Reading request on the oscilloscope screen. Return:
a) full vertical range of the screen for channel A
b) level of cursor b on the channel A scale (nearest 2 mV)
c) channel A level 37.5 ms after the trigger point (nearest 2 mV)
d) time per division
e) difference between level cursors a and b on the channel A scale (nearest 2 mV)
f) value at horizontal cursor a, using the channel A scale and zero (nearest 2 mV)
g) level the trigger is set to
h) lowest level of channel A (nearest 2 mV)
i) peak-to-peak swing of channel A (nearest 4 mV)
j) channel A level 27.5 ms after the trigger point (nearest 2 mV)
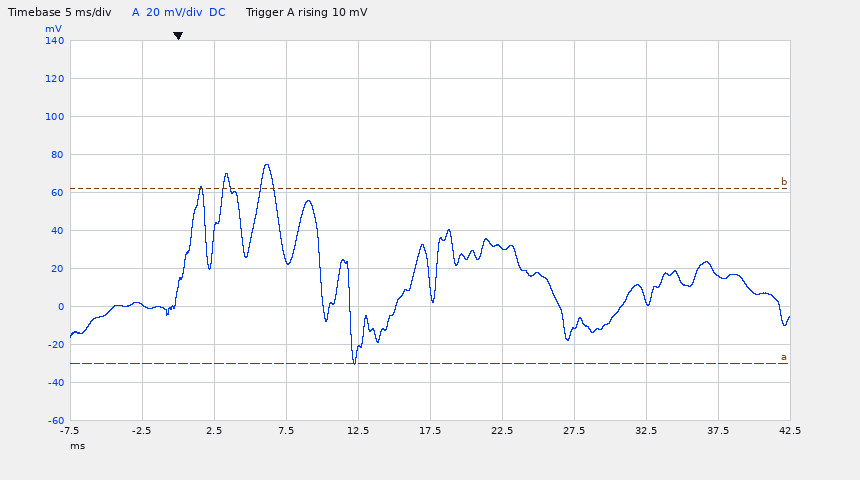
200 mV
62 mV
16 mV
5 ms
92 mV
-30 mV
10 mV
-30 mV
104 mV
-12 mV
